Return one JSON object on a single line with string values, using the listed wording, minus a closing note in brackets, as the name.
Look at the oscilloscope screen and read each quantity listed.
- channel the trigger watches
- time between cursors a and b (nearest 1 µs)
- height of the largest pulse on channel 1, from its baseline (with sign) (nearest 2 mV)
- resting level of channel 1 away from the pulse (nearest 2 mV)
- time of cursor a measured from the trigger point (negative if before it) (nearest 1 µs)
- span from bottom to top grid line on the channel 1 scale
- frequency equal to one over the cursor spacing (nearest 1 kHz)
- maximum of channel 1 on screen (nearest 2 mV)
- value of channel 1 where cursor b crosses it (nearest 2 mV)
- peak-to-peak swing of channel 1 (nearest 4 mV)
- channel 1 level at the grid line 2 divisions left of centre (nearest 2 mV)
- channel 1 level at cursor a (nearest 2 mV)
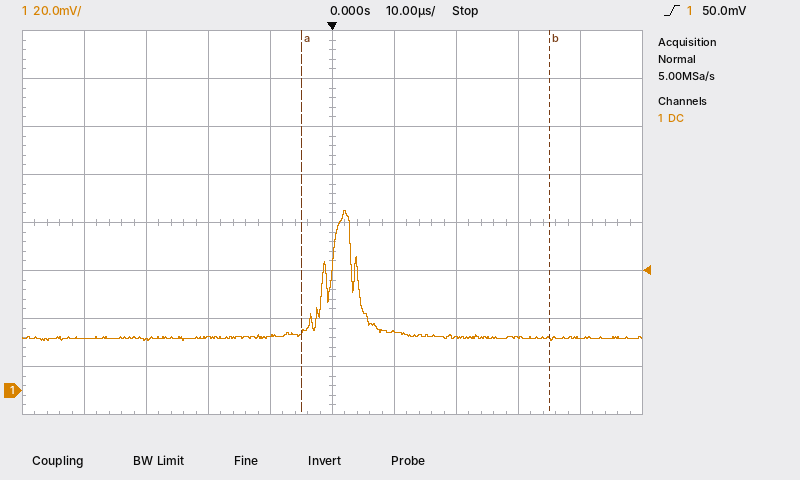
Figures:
{"channel the trigger watches": "channel 1", "time between cursors a and b": "40 µs", "height of the largest pulse on channel 1, from its baseline (with sign)": "+54 mV", "resting level of channel 1 away from the pulse": "22 mV", "time of cursor a measured from the trigger point (negative if before it)": "-5 µs", "span from bottom to top grid line on the channel 1 scale": "160 mV", "frequency equal to one over the cursor spacing": "25 kHz", "maximum of channel 1 on screen": "76 mV", "value of channel 1 where cursor b crosses it": "22 mV", "peak-to-peak swing of channel 1": "56 mV", "channel 1 level at the grid line 2 divisions left of centre": "22 mV", "channel 1 level at cursor a": "24 mV"}
